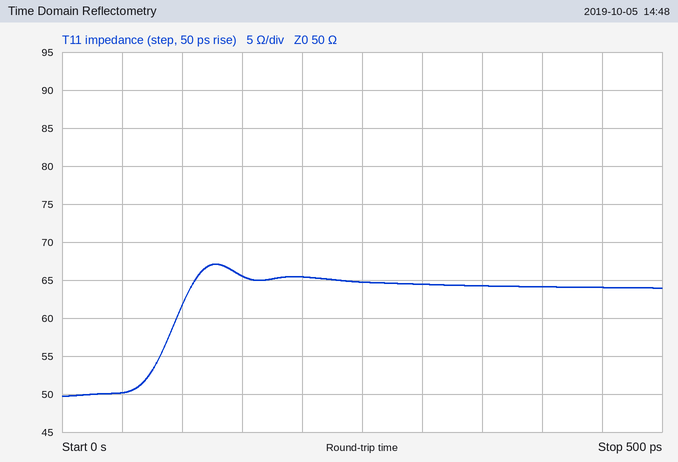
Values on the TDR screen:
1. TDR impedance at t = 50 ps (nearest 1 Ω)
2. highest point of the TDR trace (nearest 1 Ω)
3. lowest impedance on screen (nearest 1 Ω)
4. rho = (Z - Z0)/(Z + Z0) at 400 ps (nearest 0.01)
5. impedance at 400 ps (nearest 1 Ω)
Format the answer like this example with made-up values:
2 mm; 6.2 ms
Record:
50 Ω; 67 Ω; 50 Ω; +0.12; 64 Ω
